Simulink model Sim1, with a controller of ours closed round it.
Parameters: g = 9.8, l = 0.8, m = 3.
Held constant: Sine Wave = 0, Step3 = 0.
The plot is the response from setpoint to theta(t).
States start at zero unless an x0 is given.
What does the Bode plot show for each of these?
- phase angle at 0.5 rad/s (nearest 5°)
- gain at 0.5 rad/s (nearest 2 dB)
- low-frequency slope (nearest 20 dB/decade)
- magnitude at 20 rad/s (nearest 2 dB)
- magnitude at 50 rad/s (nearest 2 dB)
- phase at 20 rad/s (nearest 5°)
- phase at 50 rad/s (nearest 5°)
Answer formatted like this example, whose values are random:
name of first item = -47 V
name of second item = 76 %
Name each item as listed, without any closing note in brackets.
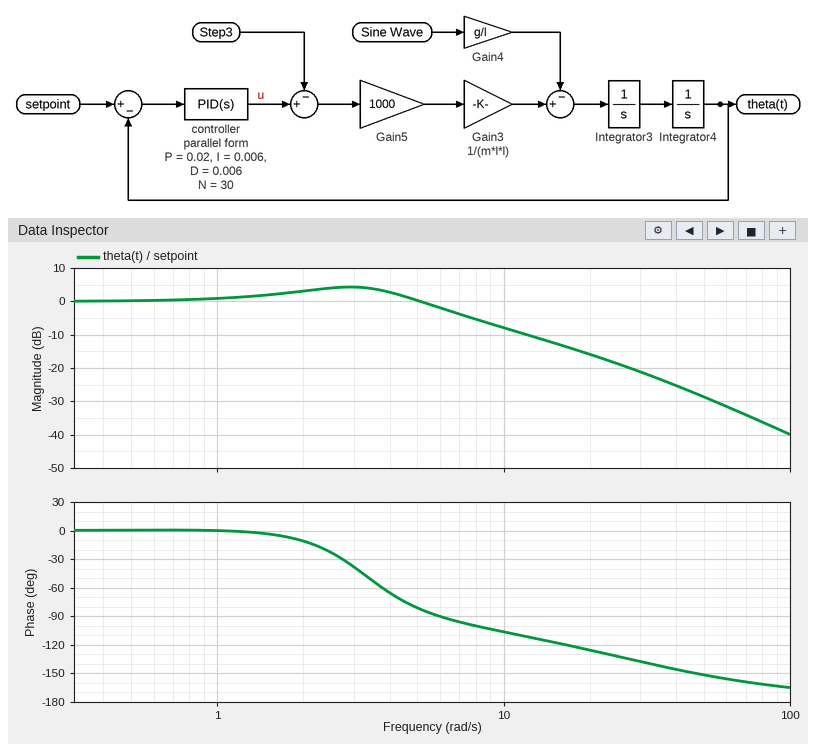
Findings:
phase angle at 0.5 rad/s = 0°
gain at 0.5 rad/s = 0 dB
low-frequency slope = 0 dB/decade
magnitude at 20 rad/s = -16 dB
magnitude at 50 rad/s = -28 dB
phase at 20 rad/s = -125°
phase at 50 rad/s = -150°
